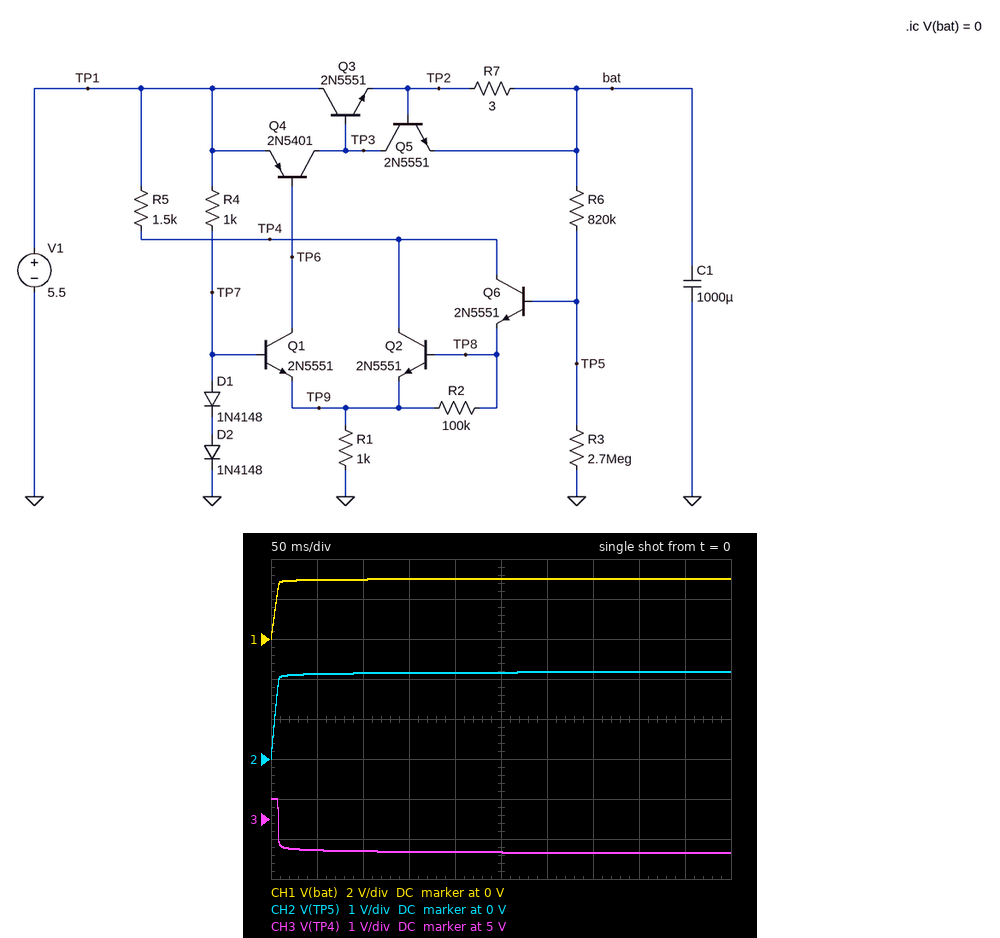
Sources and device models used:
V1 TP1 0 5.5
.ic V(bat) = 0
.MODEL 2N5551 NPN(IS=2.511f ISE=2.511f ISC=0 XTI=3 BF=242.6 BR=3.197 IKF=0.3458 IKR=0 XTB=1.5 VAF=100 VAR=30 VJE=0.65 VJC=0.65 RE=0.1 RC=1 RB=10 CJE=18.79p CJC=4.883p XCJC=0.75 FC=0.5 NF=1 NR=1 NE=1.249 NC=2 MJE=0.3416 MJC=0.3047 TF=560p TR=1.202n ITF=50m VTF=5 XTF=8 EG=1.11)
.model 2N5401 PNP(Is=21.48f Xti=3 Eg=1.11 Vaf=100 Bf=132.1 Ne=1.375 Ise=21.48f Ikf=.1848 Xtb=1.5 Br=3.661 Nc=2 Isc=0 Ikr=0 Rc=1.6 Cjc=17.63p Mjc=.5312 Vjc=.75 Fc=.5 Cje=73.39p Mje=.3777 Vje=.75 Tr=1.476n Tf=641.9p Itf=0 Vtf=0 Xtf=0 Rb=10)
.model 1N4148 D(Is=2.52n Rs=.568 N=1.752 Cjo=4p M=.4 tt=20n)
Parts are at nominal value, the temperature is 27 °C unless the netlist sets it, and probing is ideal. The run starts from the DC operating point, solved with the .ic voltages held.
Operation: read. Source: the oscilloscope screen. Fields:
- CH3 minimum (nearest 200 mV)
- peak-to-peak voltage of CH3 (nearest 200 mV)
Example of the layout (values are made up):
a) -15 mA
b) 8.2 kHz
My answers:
a) 4.2 V
b) 1.4 V
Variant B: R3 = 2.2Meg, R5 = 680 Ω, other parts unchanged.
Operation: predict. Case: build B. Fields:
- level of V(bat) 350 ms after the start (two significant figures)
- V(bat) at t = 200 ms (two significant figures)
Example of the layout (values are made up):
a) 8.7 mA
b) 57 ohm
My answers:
a) 3.2 V
b) 3.1 V
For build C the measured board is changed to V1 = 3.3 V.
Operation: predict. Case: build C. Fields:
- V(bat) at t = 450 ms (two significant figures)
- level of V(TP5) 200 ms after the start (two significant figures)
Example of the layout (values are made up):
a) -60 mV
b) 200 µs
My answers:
a) 2.7 V
b) 1.9 V
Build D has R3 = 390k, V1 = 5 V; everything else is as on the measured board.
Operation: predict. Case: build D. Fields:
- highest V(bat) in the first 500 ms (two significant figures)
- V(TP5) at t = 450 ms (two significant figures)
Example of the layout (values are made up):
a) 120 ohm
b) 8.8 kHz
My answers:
a) 4.4 V
b) 1.4 V
